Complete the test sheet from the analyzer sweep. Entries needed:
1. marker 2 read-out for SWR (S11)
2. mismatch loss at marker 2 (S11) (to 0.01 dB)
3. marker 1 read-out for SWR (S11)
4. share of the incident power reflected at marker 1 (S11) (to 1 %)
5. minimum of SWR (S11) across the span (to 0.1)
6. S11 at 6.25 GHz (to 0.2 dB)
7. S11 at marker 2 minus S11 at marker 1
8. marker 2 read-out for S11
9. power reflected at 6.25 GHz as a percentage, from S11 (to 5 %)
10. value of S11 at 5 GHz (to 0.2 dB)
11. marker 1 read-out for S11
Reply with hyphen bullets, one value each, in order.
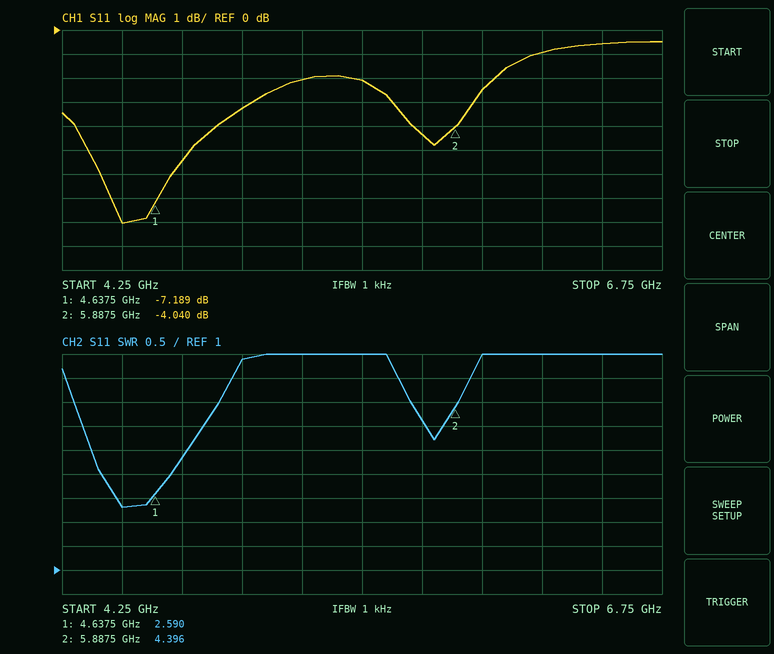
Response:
- 4.396
- 2.18 dB
- 2.590
- 19 %
- 2.3
- -1.0 dB
- 3.149 dB
- -4.040 dB
- 80 %
- -3.2 dB
- -7.189 dB
